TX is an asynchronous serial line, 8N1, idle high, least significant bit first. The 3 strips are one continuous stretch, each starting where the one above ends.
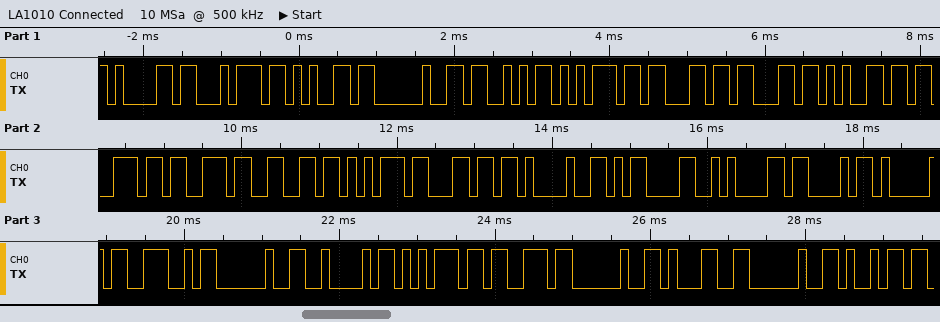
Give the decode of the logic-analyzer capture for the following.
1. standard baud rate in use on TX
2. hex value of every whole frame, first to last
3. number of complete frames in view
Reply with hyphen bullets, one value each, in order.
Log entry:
- 9600 baud
- 0x61 0x74 0x65 0x20 0x53 0x75 0x63 0x63 0x65 0x73 0x73 0x66 0x75 0x6C 0x21 0x0D 0x0A 0x43 0x41 0x4E 0x20 0x42 0x75 0x73 0x20 0x31 0x20 0x69
- 28
